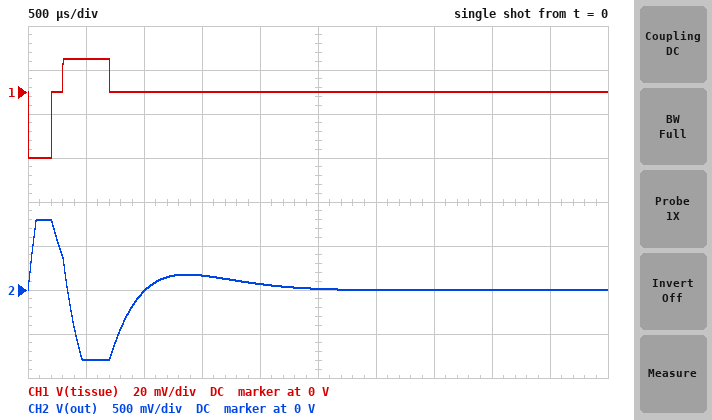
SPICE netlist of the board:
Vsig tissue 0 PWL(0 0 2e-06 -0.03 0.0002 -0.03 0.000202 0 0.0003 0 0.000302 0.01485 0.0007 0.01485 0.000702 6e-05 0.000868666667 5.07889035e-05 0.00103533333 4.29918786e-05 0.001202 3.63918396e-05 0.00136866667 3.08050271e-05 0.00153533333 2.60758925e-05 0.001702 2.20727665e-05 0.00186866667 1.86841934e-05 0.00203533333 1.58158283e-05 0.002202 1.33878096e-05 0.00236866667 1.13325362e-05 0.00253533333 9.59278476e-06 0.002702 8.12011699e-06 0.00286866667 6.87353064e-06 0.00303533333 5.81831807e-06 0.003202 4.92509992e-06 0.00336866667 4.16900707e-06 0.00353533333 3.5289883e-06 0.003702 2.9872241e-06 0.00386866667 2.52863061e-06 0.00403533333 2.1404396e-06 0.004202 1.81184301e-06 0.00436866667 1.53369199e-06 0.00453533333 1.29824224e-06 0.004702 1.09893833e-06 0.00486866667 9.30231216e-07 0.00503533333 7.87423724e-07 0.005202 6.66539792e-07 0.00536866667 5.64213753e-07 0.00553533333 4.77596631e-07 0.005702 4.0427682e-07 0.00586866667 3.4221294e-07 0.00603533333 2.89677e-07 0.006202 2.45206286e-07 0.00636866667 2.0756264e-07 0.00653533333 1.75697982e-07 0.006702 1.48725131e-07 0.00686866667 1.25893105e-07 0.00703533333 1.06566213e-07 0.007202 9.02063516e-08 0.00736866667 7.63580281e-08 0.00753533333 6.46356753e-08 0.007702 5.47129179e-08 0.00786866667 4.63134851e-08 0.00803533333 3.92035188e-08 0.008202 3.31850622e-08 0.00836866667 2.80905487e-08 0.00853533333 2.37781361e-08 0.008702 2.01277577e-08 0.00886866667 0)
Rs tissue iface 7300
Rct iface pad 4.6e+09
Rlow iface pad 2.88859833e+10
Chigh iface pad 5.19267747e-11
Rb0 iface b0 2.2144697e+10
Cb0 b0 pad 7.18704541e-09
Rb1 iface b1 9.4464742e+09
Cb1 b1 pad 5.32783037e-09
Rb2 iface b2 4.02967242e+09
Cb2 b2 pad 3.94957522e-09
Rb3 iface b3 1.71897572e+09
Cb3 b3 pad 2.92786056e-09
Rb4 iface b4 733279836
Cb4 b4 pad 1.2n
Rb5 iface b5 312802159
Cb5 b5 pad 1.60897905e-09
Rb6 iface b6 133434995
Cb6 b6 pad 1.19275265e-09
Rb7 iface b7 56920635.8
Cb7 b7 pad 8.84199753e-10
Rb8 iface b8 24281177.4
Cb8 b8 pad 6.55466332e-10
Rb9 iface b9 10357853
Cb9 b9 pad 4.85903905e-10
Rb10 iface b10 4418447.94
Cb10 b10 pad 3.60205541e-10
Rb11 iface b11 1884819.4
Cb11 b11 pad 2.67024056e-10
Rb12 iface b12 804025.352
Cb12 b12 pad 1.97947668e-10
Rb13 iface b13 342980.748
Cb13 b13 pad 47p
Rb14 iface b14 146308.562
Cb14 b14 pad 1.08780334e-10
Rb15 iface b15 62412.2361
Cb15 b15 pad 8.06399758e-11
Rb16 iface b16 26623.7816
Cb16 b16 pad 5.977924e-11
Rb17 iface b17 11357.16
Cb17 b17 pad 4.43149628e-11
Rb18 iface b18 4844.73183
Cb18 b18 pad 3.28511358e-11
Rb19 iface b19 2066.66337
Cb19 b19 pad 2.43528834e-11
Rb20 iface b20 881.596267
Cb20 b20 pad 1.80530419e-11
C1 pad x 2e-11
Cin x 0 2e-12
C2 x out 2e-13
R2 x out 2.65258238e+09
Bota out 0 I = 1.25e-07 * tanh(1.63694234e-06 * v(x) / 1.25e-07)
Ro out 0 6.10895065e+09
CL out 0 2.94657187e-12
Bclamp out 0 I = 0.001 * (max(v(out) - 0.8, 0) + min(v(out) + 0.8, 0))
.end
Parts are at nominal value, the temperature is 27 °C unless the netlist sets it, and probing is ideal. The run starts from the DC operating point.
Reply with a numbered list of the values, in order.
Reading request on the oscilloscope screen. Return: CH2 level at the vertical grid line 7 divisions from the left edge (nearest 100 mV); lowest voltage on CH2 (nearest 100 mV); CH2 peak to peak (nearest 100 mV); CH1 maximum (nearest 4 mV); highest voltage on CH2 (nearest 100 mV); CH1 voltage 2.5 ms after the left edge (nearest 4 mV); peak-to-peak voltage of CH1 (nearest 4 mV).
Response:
1. 0 V
2. -800 mV
3. 1.6 V
4. 16 mV
5. 800 mV
6. 0 V
7. 44 mV
